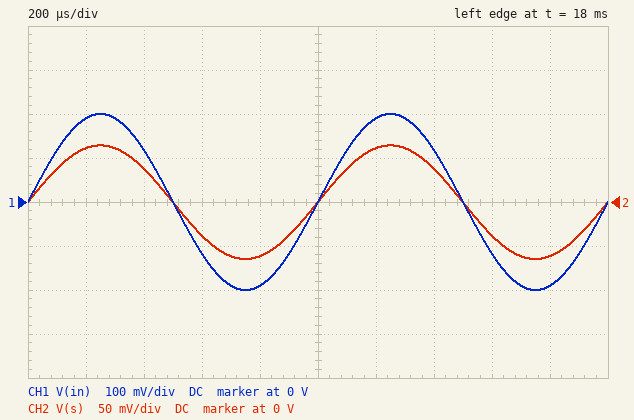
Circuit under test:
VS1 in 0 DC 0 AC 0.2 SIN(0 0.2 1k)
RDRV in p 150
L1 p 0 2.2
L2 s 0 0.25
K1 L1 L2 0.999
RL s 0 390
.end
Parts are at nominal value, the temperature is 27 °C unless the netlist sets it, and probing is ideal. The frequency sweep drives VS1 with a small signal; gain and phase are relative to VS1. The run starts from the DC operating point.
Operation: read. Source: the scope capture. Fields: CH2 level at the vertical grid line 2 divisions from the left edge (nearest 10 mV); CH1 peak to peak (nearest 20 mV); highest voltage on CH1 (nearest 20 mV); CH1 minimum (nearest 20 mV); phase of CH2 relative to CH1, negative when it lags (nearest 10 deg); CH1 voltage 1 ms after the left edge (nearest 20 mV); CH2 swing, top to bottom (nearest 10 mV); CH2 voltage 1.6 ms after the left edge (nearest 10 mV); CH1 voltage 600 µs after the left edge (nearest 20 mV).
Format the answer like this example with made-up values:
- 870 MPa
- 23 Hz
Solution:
- 40 mV
- 400 mV
- 200 mV
- -200 mV
- 0 deg
- 0 V
- 130 mV
- -40 mV
- -120 mV
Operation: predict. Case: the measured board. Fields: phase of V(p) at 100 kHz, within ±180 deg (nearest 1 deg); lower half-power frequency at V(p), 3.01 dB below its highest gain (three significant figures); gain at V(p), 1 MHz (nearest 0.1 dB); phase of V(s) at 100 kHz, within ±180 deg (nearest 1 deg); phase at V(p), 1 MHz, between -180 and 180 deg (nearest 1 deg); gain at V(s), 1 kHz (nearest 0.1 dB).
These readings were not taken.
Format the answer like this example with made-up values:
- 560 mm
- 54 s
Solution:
- 1 deg
- 11.4 Hz
- 0 dB
- -38 deg
- 0 deg
- -9.8 dB
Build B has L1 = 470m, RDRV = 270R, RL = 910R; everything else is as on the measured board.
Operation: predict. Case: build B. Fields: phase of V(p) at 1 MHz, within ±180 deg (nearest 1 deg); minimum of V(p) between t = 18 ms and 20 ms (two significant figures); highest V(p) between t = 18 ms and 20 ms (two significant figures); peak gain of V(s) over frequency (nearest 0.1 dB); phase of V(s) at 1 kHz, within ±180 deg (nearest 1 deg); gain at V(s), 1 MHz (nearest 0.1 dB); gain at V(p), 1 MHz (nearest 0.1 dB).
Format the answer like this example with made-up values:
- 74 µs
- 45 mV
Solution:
- 2 deg
- -170 mV
- 170 mV
- -4.0 dB
- 4 deg
- -14.0 dB
- -0.1 dB
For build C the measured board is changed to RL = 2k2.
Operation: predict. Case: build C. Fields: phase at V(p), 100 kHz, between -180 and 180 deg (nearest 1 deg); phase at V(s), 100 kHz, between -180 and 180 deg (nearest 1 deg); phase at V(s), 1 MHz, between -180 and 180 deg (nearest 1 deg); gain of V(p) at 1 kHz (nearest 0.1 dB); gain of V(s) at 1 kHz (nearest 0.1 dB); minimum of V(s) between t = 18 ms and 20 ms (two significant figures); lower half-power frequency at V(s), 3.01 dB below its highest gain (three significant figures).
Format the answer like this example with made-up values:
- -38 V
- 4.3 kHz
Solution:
- 0 deg
- -8 deg
- -55 deg
- -0.1 dB
- -9.5 dB
- -67 mV
- 10.8 Hz
